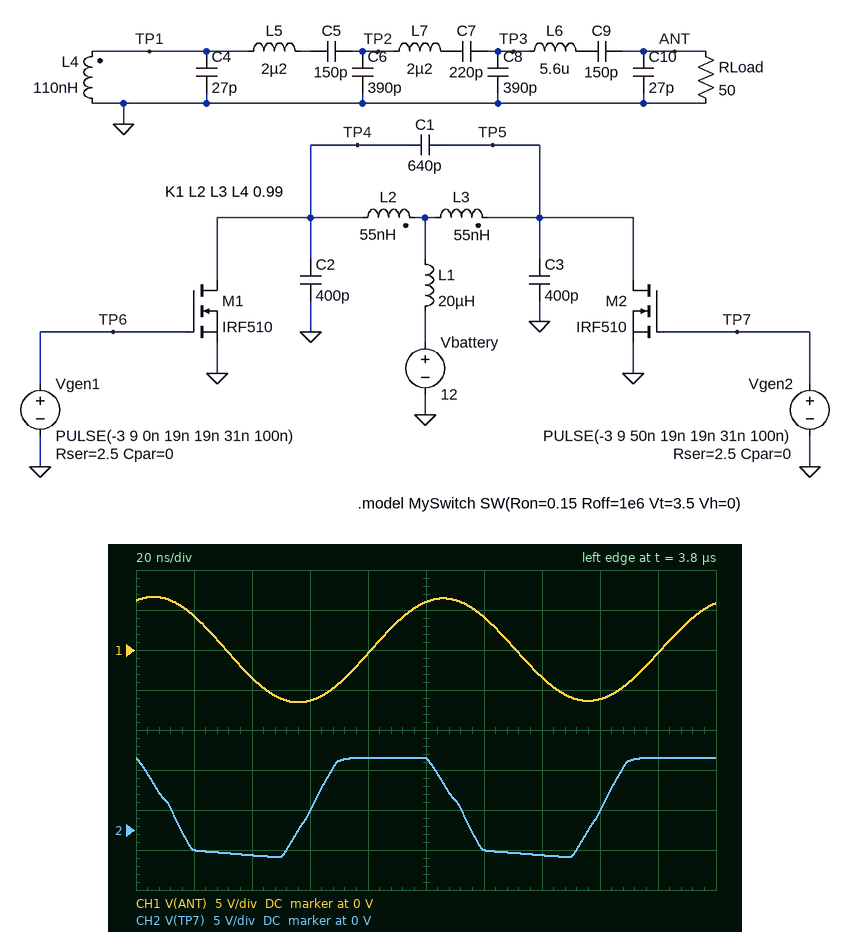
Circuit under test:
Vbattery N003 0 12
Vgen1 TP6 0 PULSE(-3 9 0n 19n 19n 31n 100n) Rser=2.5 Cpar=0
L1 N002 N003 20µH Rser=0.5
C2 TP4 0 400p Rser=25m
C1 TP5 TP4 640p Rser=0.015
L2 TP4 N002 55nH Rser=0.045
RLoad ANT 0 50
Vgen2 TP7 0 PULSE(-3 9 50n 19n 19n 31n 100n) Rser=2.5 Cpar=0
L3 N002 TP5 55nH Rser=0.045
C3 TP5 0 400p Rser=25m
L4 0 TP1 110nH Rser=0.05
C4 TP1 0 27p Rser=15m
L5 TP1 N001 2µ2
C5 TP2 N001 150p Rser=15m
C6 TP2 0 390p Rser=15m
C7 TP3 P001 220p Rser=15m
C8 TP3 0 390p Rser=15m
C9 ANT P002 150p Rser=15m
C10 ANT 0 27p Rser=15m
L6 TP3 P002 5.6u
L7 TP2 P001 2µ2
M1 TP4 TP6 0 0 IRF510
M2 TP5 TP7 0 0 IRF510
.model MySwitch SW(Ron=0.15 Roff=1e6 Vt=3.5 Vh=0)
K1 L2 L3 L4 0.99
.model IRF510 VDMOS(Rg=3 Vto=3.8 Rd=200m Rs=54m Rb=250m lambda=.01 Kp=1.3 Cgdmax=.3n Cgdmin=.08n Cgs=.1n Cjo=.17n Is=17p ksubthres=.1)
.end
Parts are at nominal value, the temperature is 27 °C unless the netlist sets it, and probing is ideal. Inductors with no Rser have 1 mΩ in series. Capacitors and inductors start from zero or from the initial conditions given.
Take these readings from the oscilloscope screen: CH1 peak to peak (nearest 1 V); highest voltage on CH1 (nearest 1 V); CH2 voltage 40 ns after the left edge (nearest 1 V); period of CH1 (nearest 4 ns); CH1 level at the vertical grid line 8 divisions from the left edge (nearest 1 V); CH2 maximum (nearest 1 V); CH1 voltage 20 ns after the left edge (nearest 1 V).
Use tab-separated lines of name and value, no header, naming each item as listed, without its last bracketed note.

CH1 peak to peak	13 V
highest voltage on CH1	7 V
CH2 voltage 40 ns after the left edge	-3 V
period of CH1	100 ns
CH1 level at the vertical grid line 8 divisions from the left edge	-6 V
CH2 maximum	9 V
CH1 voltage 20 ns after the left edge	4 V
